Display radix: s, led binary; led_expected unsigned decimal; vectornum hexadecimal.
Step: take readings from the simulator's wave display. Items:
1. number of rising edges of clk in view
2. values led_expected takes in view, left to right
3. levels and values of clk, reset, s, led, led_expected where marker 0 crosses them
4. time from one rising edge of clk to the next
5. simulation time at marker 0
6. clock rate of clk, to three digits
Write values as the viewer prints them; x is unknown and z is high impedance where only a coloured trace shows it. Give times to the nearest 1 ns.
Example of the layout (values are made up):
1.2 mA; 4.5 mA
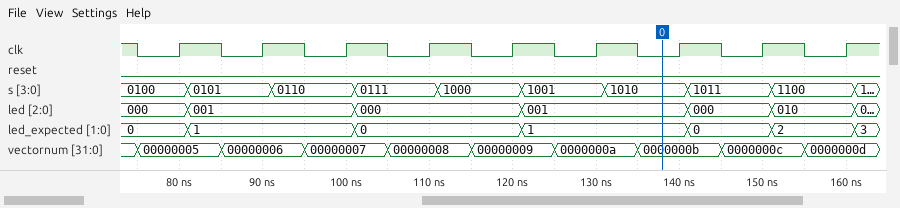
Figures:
9; 0, 1, 0, 1, 0, 2, 3; clk=0, reset=0, s=1010, led=001, led_expected=1; 10 ns; 138 ns; 100 MHz
